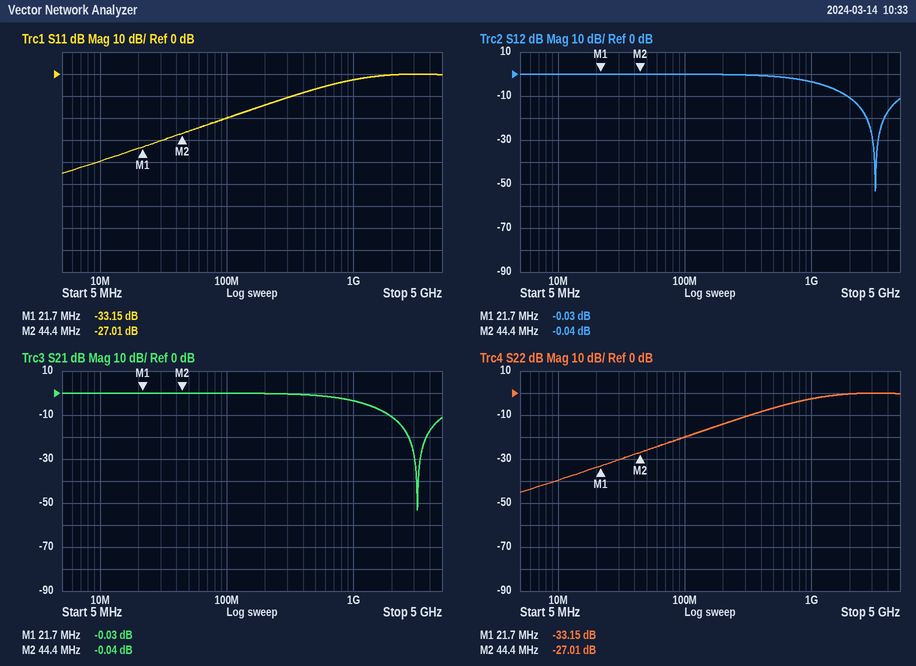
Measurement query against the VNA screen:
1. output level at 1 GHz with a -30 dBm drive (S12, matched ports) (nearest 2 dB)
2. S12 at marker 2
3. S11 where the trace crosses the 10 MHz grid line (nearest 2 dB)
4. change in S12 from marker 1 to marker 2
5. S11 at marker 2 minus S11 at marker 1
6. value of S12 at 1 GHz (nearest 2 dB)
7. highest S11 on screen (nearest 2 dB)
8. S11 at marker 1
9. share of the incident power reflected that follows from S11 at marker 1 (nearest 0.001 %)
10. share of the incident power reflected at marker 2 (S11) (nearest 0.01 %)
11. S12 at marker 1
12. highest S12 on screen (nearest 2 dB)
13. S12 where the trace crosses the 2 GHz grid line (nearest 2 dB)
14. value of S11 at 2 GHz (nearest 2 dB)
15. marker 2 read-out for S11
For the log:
-34 dBm
-0.04 dB
-40 dB
-0.01 dB
6.14 dB
-4 dB
0 dB
-33.15 dB
0.048 %
0.20 %
-0.03 dB
0 dB
-10 dB
0 dB
-27.01 dB
